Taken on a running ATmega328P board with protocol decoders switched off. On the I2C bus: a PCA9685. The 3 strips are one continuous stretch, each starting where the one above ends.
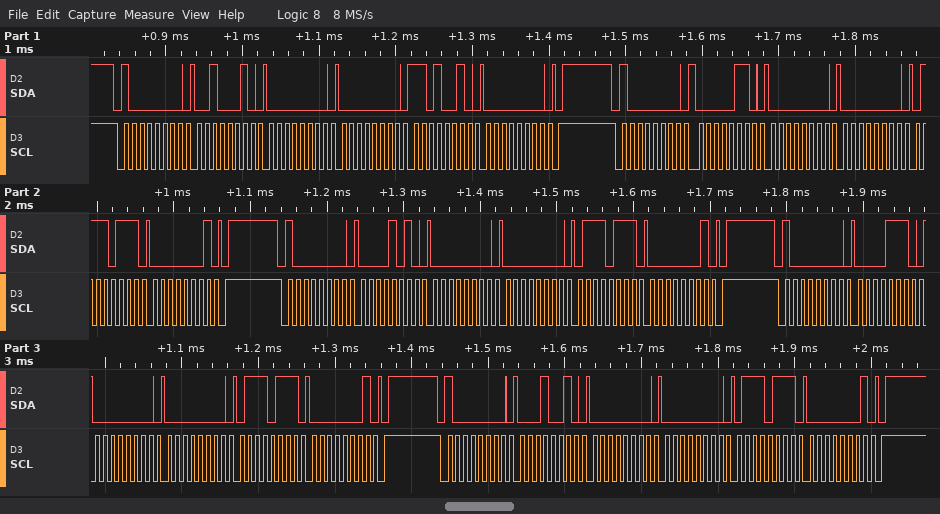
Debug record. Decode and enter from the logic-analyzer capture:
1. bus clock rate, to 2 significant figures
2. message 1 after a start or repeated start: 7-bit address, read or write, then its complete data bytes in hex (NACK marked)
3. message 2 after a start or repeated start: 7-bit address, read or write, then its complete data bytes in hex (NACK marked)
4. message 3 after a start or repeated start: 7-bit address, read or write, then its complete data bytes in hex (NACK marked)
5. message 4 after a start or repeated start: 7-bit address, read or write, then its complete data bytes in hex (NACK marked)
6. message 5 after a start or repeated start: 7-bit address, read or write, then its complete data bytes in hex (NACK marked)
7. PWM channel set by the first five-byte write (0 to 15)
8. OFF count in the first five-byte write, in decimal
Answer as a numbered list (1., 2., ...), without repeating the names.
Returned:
1. 100 kHz
2. 0x40 write: 22 00 00 D2 00
3. 0x40 write: 06 00 00 77 01
4. 0x40 write: 0A 00 00 77 01
5. 0x40 write: 0E 00 00 77 01
6. 0x40 write: 12 00 00 77 01
7. 7
8. 210
